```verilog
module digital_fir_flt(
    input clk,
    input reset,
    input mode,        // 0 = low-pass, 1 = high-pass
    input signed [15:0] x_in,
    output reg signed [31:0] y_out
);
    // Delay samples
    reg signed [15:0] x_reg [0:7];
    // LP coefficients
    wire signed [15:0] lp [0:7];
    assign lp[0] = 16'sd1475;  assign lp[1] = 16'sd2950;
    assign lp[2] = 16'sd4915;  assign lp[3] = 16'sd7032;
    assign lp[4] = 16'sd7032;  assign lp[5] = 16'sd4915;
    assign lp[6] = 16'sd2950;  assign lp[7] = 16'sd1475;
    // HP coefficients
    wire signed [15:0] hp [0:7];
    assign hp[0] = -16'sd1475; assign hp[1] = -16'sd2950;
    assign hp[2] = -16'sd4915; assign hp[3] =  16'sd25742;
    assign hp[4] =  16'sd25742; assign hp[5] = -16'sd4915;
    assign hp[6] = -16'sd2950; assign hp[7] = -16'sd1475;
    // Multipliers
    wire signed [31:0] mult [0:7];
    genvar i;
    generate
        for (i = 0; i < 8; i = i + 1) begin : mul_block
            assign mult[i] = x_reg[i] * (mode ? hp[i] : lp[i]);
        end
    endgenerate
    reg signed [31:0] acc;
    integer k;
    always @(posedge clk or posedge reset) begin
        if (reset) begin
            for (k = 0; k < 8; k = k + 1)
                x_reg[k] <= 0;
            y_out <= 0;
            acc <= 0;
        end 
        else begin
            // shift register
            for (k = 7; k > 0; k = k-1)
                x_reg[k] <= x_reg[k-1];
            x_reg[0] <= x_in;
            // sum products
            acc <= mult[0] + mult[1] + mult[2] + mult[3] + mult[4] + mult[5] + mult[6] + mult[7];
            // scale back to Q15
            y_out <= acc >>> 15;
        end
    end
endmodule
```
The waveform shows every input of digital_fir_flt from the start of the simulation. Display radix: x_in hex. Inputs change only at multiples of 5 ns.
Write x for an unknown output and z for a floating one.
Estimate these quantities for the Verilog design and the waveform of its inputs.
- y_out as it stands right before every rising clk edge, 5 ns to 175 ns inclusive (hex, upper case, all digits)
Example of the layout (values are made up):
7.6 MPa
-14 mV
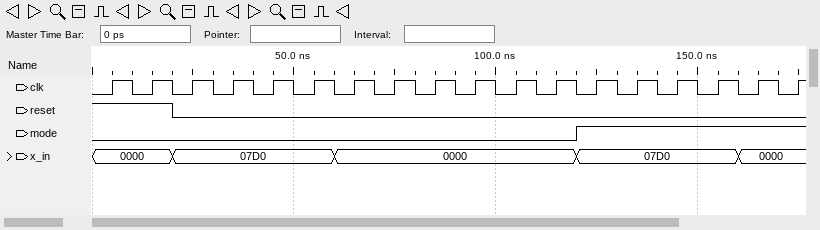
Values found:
00000000, 00000000, 00000000, 00000000, 00000000, 0000005A, 0000010E, 0000023A, 000003E7, 0000053A, 000005B2, 0000053A, 000003E7, 0000023A, FFFFFEF1, FFFFFF4B, FFFFFEF1, FFFFFDC5
